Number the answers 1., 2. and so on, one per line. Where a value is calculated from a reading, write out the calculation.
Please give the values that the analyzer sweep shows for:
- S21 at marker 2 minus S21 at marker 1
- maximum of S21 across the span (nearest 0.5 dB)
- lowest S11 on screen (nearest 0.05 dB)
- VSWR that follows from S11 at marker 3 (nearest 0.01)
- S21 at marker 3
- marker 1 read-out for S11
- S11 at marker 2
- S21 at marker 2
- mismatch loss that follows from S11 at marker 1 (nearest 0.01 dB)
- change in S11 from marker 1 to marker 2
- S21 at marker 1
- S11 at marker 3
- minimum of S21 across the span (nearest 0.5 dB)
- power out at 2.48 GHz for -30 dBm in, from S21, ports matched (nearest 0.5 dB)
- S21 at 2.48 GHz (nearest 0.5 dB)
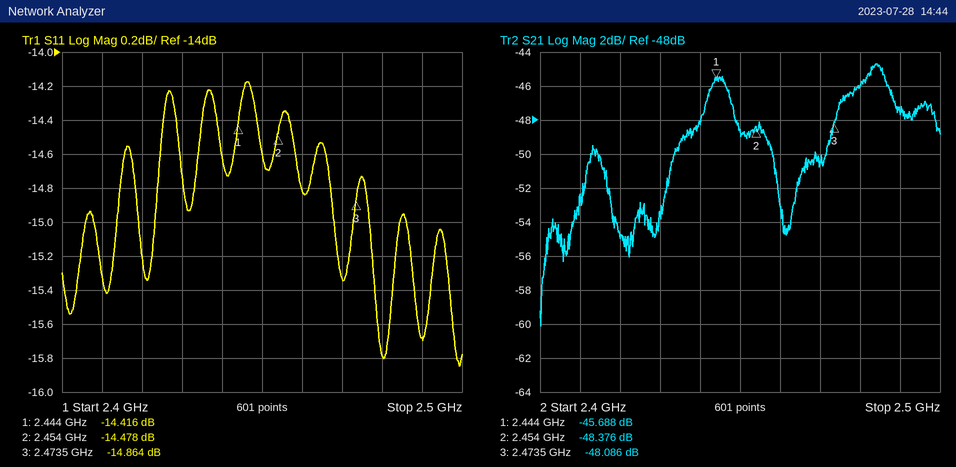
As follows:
1. -48.376 − (-45.688) = -2.688 dB
2. -44.5 dB
3. -15.85 dB
4. (1 + 0.1806)/(1 − 0.1806) ≈ 1.44
5. -48.086 dB
6. -14.416 dB
7. -14.478 dB
8. -48.376 dB
9. −10 log10(1 − 10^(-14.416/10)) ≈ 0.16 dB
10. -14.478 − (-14.416) = -0.062 dB
11. -45.688 dB
12. -14.864 dB
13. -60.0 dB
14. -30 dBm + (-46.0 dB) = -76.0 dBm
15. -46.0 dB
